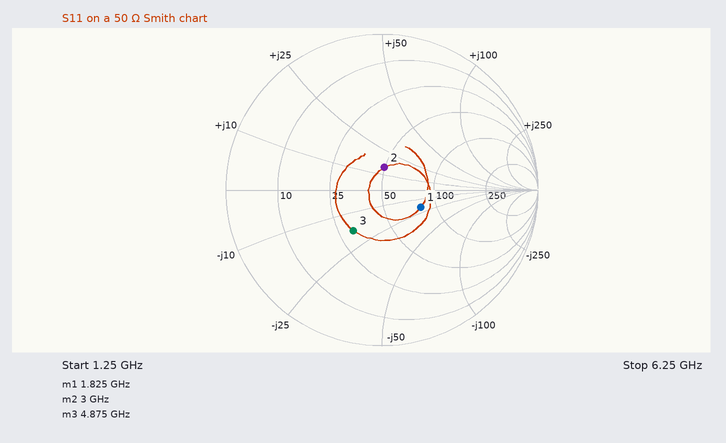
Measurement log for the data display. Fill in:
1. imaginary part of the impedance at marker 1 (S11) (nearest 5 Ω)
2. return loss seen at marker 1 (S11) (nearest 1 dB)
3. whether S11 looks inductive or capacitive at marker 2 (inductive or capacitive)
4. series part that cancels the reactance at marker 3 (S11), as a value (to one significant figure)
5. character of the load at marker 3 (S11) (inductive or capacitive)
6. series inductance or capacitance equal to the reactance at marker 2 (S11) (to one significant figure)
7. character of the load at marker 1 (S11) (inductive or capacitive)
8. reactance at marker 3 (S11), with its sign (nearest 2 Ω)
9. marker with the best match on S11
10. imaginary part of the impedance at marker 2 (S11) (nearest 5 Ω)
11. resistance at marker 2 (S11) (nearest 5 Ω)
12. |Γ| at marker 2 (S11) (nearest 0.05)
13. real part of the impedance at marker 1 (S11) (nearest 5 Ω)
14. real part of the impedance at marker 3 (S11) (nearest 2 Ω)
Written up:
-20 Ω
11 dB
inductive
600 pH
capacitive
800 pH
capacitive
-18 Ω
marker 2
+15 Ω
50 Ω
0.15
80 Ω
30 Ω
